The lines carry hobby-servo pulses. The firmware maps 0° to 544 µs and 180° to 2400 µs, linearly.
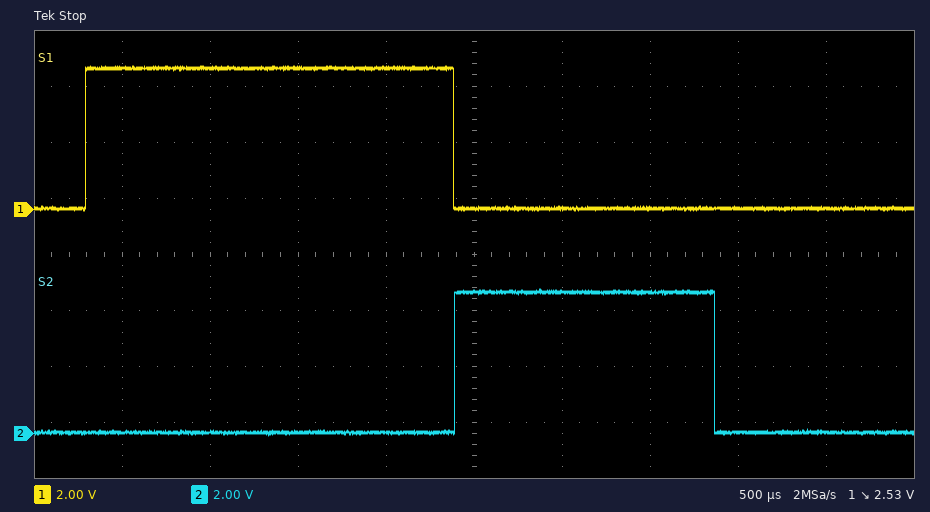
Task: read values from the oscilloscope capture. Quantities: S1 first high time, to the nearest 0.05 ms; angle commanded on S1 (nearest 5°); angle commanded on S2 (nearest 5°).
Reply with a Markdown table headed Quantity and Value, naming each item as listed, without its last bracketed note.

| Quantity | Value |
|---|---|
| S1 first high time, to the nearest 0.05 ms | 2.10 ms |
| angle commanded on S1 | 150° |
| angle commanded on S2 | 90° |
